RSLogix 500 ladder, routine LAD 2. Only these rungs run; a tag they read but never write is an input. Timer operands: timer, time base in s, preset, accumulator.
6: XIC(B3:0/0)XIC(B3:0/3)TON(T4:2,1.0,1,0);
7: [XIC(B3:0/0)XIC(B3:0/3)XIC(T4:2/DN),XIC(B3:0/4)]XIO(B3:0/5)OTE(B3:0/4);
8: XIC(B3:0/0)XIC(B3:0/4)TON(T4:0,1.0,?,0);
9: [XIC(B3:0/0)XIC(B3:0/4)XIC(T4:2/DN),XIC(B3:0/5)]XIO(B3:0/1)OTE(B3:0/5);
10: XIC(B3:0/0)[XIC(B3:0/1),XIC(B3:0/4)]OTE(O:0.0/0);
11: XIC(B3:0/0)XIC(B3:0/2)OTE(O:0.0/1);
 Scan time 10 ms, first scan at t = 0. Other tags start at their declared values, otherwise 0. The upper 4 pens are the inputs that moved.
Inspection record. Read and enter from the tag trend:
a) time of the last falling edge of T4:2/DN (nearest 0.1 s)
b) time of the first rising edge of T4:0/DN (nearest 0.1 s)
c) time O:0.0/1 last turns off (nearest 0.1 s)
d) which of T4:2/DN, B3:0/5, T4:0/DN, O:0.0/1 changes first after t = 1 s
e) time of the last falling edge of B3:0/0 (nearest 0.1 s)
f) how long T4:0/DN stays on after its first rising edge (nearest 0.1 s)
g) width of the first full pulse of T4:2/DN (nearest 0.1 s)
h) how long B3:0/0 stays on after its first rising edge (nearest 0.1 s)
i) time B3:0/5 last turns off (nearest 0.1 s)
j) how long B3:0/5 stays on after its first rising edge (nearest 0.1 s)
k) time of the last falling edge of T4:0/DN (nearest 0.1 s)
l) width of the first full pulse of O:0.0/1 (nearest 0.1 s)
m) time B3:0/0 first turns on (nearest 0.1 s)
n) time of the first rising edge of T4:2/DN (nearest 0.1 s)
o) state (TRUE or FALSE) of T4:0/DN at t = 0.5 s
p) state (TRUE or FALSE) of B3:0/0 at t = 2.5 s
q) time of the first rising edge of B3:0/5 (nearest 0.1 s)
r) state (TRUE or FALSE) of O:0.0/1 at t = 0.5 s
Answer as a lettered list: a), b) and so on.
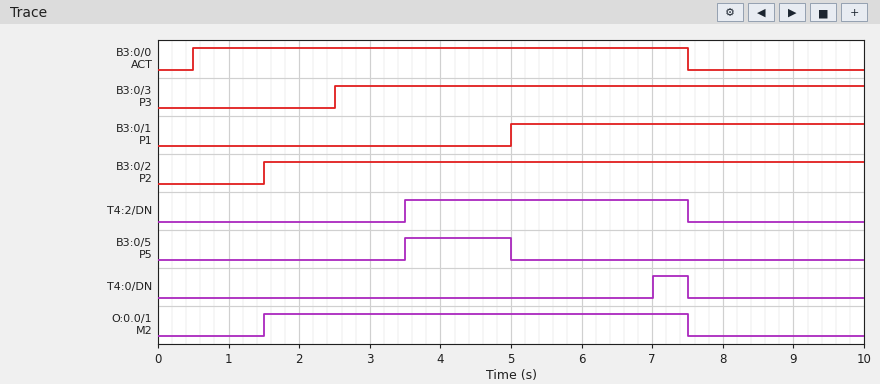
a) 7.5 s
b) 7.0 s
c) 7.5 s
d) O:0.0/1
e) 7.5 s
f) 0.5 s
g) 4.0 s
h) 7.0 s
i) 5.0 s
j) 1.5 s
k) 7.5 s
l) 6.0 s
m) 0.5 s
n) 3.5 s
o) FALSE
p) TRUE
q) 3.5 s
r) FALSE
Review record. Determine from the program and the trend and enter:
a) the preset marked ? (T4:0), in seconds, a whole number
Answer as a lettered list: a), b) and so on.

a) 2 s
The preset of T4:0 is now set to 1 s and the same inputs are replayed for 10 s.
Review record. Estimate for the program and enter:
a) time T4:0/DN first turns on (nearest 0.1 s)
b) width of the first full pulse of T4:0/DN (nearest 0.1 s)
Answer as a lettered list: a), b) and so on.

a) 6.0 s
b) 1.5 s
